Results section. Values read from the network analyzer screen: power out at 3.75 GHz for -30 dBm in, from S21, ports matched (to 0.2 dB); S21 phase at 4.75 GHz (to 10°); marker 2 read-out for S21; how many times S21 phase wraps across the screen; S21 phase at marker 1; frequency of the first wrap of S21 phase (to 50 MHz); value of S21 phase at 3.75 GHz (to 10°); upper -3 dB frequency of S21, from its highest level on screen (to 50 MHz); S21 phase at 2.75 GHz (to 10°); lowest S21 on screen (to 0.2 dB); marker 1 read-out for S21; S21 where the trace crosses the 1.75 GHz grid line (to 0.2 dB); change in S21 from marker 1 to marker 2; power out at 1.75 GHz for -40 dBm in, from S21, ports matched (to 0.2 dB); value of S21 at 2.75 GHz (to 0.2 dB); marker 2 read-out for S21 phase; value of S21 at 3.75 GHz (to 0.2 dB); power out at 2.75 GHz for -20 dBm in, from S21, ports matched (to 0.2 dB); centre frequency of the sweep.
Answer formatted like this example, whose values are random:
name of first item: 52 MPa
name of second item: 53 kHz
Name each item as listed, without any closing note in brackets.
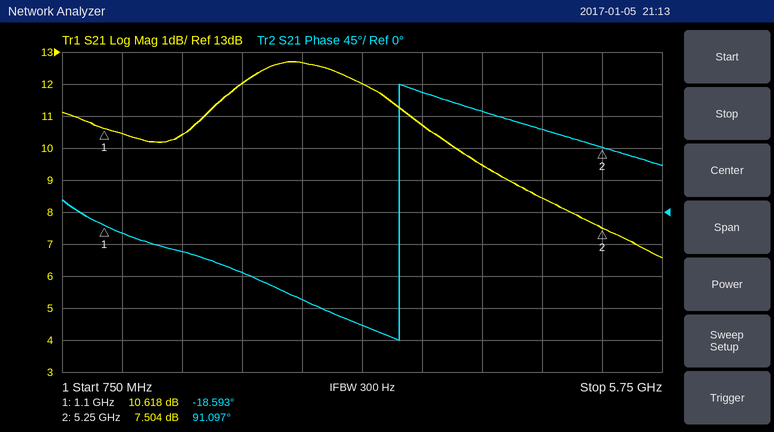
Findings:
power out at 3.75 GHz for -30 dBm in, from S21, ports matched: -19.2 dBm
S21 phase at 4.75 GHz: 120°
marker 2 read-out for S21: 7.504 dB
how many times S21 phase wraps across the screen: 1
S21 phase at marker 1: -18.593°
frequency of the first wrap of S21 phase: 3.55 GHz
value of S21 phase at 3.75 GHz: 170°
upper -3 dB frequency of S21, from its highest level on screen: 4.15 GHz
S21 phase at 2.75 GHz: -120°
lowest S21 on screen: 6.6 dB
marker 1 read-out for S21: 10.618 dB
S21 where the trace crosses the 1.75 GHz grid line: 10.4 dB
change in S21 from marker 1 to marker 2: -3.114 dB
power out at 1.75 GHz for -40 dBm in, from S21, ports matched: -29.6 dBm
value of S21 at 2.75 GHz: 12.6 dB
marker 2 read-out for S21 phase: 91.097°
value of S21 at 3.75 GHz: 10.8 dB
power out at 2.75 GHz for -20 dBm in, from S21, ports matched: -7.4 dBm
centre frequency of the sweep: 3.25 GHz
